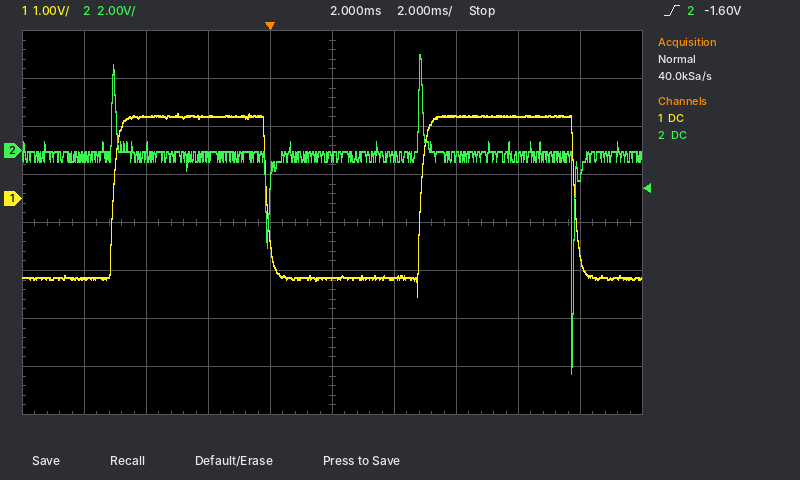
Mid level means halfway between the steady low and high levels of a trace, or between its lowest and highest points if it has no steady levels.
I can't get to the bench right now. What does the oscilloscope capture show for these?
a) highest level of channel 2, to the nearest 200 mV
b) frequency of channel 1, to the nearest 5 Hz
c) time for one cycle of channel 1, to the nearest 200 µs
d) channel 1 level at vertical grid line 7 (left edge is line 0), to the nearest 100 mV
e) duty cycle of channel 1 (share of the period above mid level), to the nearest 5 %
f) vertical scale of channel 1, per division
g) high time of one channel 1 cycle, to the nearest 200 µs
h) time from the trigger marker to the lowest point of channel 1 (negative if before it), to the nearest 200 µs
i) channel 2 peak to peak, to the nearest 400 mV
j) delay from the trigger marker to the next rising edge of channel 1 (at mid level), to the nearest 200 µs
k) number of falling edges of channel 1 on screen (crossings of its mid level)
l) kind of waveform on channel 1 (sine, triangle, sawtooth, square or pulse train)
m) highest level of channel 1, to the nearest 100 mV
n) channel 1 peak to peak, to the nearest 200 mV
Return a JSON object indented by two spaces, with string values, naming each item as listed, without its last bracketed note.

{
  "highest level of channel 2, to the nearest 200 mV": "4.0 V",
  "frequency of channel 1, to the nearest 5 Hz": "100 Hz",
  "time for one cycle of channel 1, to the nearest 200 µs": "10.0 ms",
  "channel 1 level at vertical grid line 7 (left edge is line 0), to the nearest 100 mV": "1.7 V",
  "duty cycle of channel 1 (share of the period above mid level), to the nearest 5 %": "50 %",
  "vertical scale of channel 1, per division": "1 V",
  "high time of one channel 1 cycle, to the nearest 200 µs": "5.0 ms",
  "time from the trigger marker to the lowest point of channel 1 (negative if before it), to the nearest 200 µs": "+4.8 ms",
  "channel 2 peak to peak, to the nearest 400 mV": "13.2 V",
  "delay from the trigger marker to the next rising edge of channel 1 (at mid level), to the nearest 200 µs": "4.8 ms",
  "number of falling edges of channel 1 on screen": "2",
  "kind of waveform on channel 1": "square",
  "highest level of channel 1, to the nearest 100 mV": "1.8 V",
  "channel 1 peak to peak, to the nearest 200 mV": "3.8 V"
}
